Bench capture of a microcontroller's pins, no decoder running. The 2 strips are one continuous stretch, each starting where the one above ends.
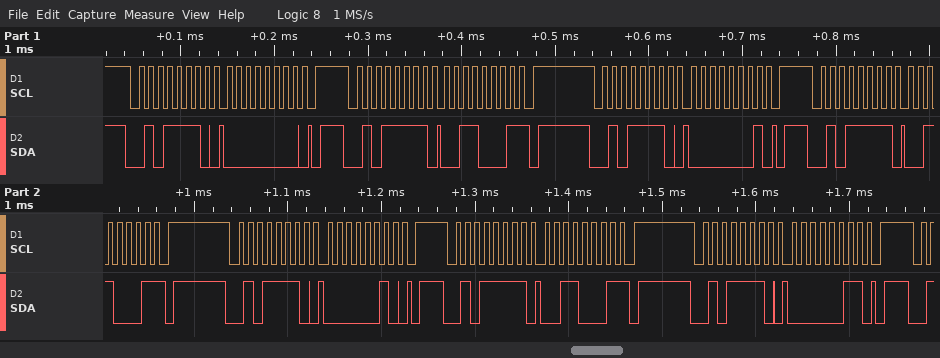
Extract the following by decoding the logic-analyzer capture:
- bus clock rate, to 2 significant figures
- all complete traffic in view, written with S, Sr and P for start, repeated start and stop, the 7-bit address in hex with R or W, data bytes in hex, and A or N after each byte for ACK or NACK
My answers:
100 kHz
S 2FW A 00 A P S 2FR A 31 N P S 2FW A 01 A P S 2FR A 31 N P S 2FW A 02 A P S 2FR A 31 N P S 2FW A 03 A P
